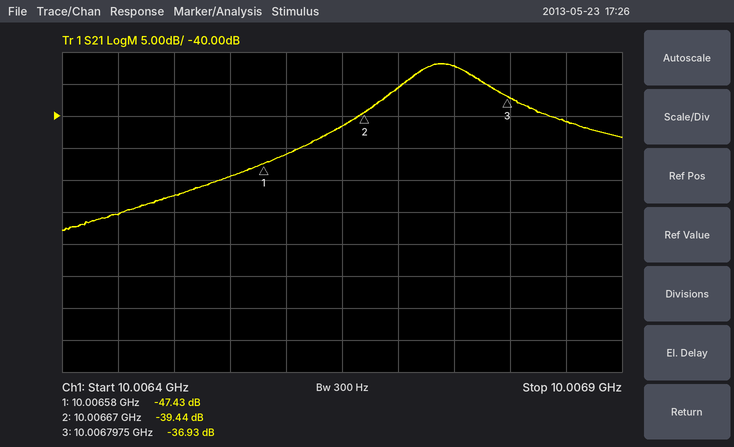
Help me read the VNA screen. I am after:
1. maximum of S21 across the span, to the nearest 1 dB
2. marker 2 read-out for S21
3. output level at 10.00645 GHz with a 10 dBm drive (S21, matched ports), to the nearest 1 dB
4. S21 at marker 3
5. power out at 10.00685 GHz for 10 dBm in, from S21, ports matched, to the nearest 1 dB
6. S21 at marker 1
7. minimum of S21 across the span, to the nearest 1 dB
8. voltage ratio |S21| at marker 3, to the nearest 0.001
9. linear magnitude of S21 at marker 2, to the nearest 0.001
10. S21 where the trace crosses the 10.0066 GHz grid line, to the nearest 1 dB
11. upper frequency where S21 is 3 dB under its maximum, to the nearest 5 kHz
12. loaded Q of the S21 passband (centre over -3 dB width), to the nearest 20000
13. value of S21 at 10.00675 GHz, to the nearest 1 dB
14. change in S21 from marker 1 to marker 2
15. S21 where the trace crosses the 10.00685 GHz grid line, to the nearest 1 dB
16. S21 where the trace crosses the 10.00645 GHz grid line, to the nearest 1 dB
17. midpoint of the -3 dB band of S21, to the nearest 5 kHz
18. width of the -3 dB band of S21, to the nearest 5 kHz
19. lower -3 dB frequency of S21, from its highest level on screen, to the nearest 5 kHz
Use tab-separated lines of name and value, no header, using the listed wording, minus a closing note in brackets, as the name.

maximum of S21 across the span, to the nearest 1 dB	-32 dB
marker 2 read-out for S21	-39.44 dB
output level at 10.00645 GHz with a 10 dBm drive (S21, matched ports), to the nearest 1 dB	-45 dBm
S21 at marker 3	-36.93 dB
power out at 10.00685 GHz for 10 dBm in, from S21, ports matched, to the nearest 1 dB	-31 dBm
S21 at marker 1	-47.43 dB
minimum of S21 across the span, to the nearest 1 dB	-58 dB
voltage ratio |S21| at marker 3, to the nearest 0.001	0.014
linear magnitude of S21 at marker 2, to the nearest 0.001	0.011
S21 where the trace crosses the 10.0066 GHz grid line, to the nearest 1 dB	-46 dB
upper frequency where S21 is 3 dB under its maximum, to the nearest 5 kHz	10.006775 GHz
loaded Q of the S21 passband (centre over -3 dB width), to the nearest 20000	140000
value of S21 at 10.00675 GHz, to the nearest 1 dB	-32 dB
change in S21 from marker 1 to marker 2	7.99 dB
S21 where the trace crosses the 10.00685 GHz grid line, to the nearest 1 dB	-41 dB
S21 where the trace crosses the 10.00645 GHz grid line, to the nearest 1 dB	-55 dB
midpoint of the -3 dB band of S21, to the nearest 5 kHz	10.006740 GHz
width of the -3 dB band of S21, to the nearest 5 kHz	70 kHz
lower -3 dB frequency of S21, from its highest level on screen, to the nearest 5 kHz	10.006705 GHz
